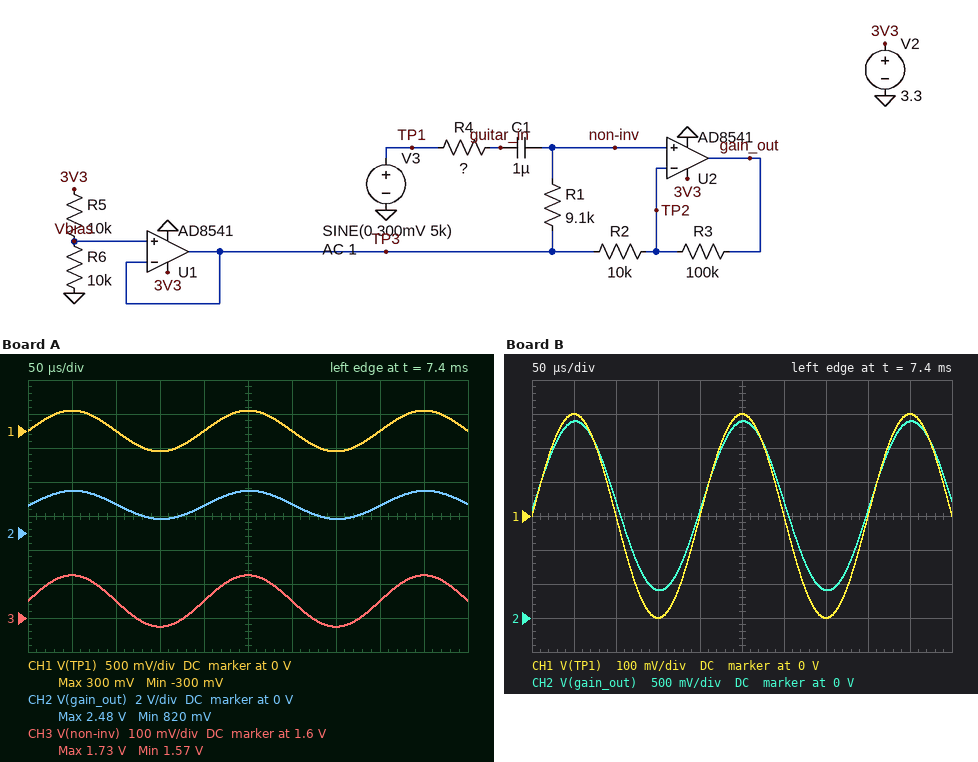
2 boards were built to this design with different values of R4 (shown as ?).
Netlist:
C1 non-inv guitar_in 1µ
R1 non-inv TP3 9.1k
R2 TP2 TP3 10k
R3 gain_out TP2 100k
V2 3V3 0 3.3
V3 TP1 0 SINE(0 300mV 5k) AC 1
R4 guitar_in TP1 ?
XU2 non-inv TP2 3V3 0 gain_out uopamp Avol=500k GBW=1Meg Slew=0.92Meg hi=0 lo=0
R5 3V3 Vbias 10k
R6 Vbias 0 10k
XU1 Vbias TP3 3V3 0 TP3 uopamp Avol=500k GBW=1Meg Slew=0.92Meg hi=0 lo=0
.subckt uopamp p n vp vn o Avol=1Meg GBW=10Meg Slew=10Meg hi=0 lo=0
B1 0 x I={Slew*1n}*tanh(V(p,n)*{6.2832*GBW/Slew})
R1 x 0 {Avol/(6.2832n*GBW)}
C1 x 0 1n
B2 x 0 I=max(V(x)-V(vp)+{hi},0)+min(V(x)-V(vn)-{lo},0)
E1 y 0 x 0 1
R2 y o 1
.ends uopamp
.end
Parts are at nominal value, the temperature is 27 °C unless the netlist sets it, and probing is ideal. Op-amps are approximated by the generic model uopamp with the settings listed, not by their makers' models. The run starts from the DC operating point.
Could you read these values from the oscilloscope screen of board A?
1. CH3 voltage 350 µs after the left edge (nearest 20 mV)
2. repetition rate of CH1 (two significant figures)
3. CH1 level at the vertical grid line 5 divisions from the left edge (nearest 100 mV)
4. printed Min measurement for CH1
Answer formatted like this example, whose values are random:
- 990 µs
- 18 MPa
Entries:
- 1.58 V
- 5.0 kHz
- 300 mV
- -300 mV
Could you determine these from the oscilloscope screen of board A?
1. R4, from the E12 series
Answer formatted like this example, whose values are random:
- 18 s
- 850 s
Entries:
- 27 kΩ
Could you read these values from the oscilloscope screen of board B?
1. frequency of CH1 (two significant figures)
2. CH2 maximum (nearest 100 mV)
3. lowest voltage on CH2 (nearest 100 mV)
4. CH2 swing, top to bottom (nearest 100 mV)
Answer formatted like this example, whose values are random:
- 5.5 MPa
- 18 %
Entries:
- 5.0 kHz
- 2.9 V
- 400 mV
- 2.5 V
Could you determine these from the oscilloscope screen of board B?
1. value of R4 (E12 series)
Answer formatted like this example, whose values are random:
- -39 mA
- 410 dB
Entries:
- 15 kΩ
